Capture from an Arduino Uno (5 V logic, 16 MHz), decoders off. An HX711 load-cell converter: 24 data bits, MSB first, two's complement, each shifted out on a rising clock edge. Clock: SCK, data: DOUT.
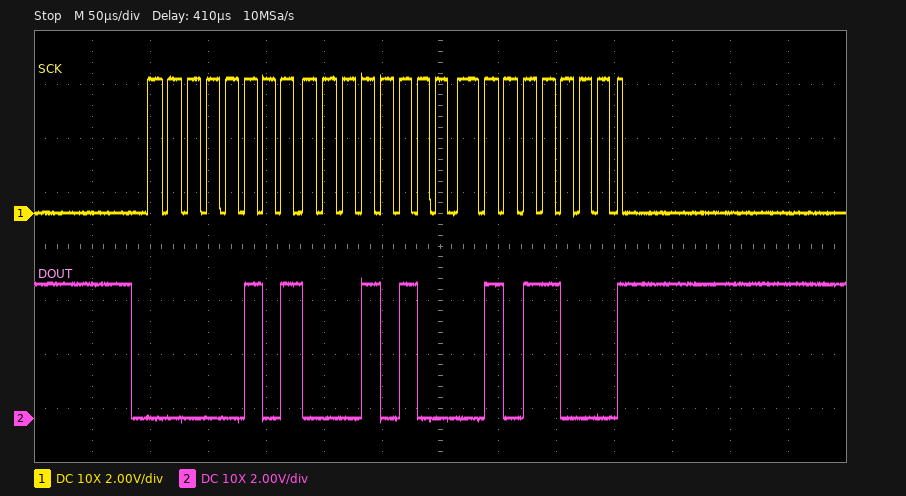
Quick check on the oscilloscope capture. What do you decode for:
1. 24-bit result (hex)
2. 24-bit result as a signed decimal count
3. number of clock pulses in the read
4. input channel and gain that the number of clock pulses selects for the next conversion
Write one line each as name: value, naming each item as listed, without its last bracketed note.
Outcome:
24-bit result: 0x051458
24-bit result as a signed decimal count: 332888
number of clock pulses in the read: 25
input channel and gain that the number of clock pulses selects for the next conversion: channel A, gain 128
